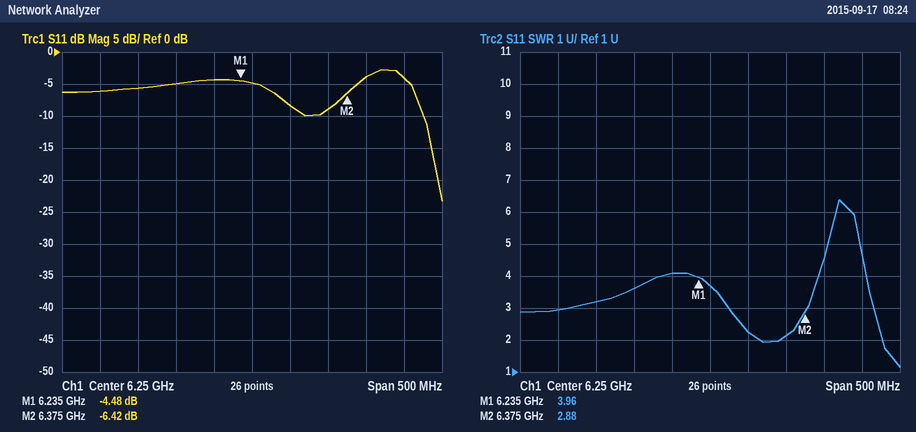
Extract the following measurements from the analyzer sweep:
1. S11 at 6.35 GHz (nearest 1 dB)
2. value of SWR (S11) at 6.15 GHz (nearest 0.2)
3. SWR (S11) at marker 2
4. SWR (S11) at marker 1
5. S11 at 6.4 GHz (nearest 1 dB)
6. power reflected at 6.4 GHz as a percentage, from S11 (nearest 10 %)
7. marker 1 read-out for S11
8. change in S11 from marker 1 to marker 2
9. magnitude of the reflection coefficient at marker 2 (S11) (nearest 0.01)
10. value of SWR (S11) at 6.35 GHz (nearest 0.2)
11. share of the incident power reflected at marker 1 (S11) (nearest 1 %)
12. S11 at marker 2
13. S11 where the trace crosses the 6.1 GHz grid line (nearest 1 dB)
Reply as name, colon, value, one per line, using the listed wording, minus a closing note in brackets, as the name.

S11 at 6.35 GHz: -9 dB
value of SWR (S11) at 6.15 GHz: 3.6
SWR (S11) at marker 2: 2.88
SWR (S11) at marker 1: 3.96
S11 at 6.4 GHz: -4 dB
power reflected at 6.4 GHz as a percentage, from S11: 40 %
marker 1 read-out for S11: -4.48 dB
change in S11 from marker 1 to marker 2: -1.94 dB
magnitude of the reflection coefficient at marker 2 (S11): 0.48
value of SWR (S11) at 6.35 GHz: 2.2
share of the incident power reflected at marker 1 (S11): 36 %
S11 at marker 2: -6.42 dB
S11 where the trace crosses the 6.1 GHz grid line: -6 dB
